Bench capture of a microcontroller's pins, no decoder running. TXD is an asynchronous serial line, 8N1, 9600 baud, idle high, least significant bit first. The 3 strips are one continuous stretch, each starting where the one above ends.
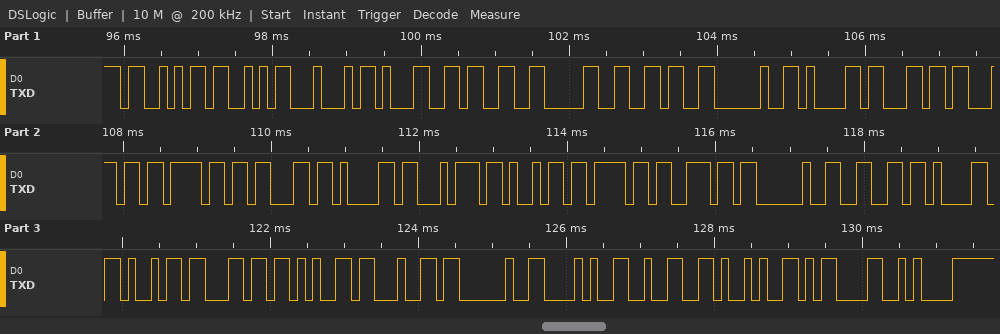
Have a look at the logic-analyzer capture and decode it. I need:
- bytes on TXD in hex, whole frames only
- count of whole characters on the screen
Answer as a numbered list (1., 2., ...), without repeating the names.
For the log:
1. 53 53 44 31 33 30 36 20 61 6C 6C 6F 63 61 74 69 6F 6E 20 66 61 69 6C 65 64 20 28 32 29 0D 0A
2. 31
